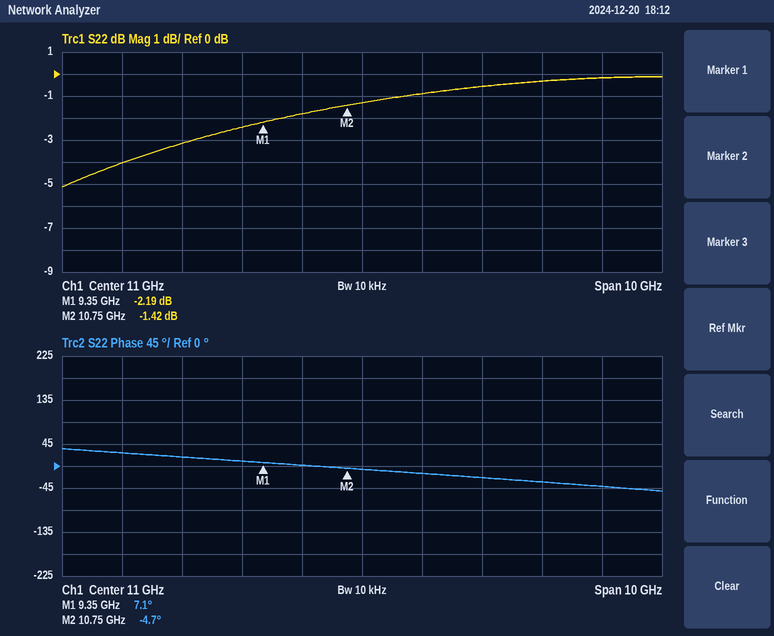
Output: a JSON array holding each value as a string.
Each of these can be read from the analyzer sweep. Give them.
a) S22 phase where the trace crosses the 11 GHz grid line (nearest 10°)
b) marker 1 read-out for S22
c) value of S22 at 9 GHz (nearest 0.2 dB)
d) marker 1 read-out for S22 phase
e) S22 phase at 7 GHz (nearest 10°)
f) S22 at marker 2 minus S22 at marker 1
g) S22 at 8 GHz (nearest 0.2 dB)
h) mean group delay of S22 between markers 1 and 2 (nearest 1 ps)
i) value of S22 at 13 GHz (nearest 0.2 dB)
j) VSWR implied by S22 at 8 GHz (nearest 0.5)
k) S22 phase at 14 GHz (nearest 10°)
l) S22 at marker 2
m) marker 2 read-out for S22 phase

["-10°", "-2.19 dB", "-2.4 dB", "7.1°", "30°", "0.77 dB", "-3.2 dB", "23 ps", "-0.6 dB", "5.5", "-30°", "-1.42 dB", "-4.7°"]
